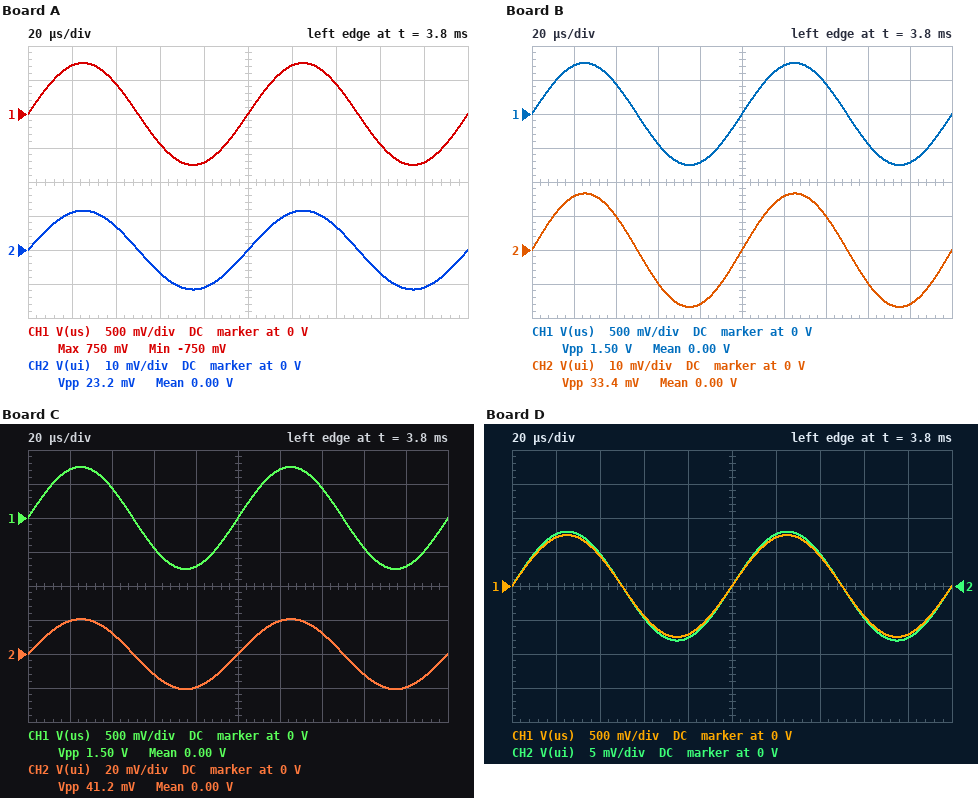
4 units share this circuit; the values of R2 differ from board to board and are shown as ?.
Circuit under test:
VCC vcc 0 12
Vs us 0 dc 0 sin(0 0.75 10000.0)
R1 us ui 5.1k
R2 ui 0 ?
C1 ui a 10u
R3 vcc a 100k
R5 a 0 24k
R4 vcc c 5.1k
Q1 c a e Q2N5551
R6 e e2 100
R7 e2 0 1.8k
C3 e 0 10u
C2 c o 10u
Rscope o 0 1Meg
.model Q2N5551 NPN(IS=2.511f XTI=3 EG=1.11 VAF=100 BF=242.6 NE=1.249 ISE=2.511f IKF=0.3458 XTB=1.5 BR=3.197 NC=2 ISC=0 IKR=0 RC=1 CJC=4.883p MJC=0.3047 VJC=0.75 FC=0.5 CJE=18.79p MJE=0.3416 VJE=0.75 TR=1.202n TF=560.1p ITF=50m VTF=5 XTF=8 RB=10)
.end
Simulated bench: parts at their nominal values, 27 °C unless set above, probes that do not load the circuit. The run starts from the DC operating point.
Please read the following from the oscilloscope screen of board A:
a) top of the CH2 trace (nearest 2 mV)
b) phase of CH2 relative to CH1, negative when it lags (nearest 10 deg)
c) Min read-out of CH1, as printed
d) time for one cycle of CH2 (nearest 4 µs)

12 mV
0 deg
-750 mV
100 µs
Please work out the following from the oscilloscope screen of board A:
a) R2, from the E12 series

82 Ω
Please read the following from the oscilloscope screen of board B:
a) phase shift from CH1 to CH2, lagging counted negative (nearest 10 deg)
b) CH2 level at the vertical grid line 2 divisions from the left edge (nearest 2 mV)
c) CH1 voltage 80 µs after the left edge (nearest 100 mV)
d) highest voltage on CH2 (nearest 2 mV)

0 deg
10 mV
-700 mV
16 mV
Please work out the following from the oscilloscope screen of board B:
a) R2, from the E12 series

120 Ω
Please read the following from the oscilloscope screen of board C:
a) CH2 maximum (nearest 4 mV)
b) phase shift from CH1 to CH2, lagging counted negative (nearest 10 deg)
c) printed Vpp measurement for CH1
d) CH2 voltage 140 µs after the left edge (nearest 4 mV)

20 mV
0 deg
1.50 V
12 mV
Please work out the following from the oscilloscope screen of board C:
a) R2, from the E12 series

150 Ω
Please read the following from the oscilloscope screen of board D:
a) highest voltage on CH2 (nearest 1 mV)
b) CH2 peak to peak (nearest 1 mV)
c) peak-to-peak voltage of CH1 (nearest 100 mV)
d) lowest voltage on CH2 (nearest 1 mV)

8 mV
16 mV
1.5 V
-8 mV
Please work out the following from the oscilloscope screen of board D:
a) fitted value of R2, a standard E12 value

56 Ω
